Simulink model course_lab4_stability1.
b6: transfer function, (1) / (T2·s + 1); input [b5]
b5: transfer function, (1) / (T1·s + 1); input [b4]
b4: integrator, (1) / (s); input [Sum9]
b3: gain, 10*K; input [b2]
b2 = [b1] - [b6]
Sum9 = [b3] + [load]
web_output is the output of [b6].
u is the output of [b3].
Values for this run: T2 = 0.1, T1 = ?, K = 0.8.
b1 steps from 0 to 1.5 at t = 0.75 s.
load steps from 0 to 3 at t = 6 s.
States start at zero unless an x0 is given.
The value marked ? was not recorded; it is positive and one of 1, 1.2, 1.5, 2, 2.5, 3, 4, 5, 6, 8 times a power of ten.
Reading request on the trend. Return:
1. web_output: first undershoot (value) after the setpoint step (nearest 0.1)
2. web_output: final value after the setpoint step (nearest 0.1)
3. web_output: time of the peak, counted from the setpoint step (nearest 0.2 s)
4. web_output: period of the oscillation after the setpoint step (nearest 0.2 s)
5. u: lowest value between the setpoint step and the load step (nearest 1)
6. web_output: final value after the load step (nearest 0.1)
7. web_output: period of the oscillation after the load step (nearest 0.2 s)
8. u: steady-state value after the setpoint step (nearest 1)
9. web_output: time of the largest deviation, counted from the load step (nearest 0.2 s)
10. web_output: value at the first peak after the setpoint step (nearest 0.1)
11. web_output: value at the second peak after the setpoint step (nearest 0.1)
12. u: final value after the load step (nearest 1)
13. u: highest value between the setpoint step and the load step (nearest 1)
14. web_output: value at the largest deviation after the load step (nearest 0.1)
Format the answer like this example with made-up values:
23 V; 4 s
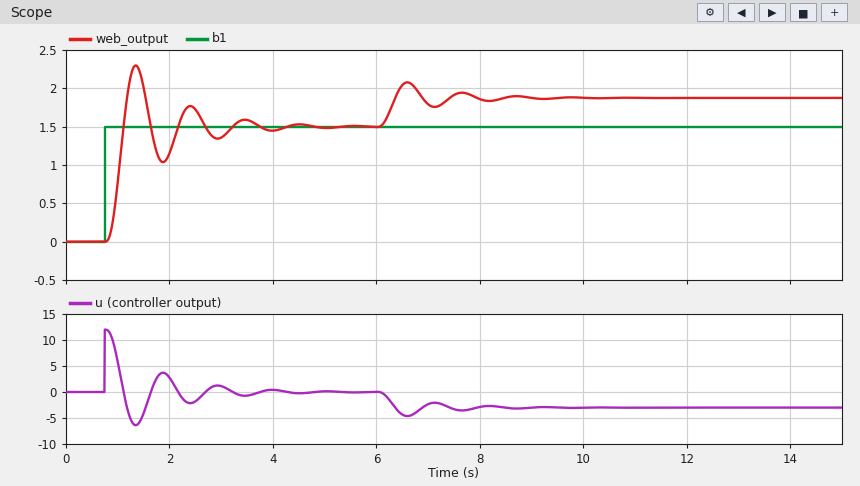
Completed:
1.0; 1.5; 0.6 s; 1.0 s; -6; 1.9; 1.0 s; 0; 0.6 s; 2.3; 1.8; -3; 12; 2.1
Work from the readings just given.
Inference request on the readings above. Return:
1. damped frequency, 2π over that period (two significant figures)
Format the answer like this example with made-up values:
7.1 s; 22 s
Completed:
6.3 rad/s
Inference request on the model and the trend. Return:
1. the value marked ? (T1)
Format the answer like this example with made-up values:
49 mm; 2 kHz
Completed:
0.15
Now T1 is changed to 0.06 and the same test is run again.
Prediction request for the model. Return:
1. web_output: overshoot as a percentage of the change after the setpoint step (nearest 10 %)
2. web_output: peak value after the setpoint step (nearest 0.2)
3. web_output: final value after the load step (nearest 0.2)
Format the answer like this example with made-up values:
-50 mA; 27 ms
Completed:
30 %; 2.0; 1.8
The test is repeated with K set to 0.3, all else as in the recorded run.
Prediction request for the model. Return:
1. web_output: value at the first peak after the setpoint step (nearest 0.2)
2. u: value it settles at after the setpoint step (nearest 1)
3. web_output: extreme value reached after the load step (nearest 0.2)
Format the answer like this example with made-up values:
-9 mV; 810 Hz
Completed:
1.8; 0; 2.6
